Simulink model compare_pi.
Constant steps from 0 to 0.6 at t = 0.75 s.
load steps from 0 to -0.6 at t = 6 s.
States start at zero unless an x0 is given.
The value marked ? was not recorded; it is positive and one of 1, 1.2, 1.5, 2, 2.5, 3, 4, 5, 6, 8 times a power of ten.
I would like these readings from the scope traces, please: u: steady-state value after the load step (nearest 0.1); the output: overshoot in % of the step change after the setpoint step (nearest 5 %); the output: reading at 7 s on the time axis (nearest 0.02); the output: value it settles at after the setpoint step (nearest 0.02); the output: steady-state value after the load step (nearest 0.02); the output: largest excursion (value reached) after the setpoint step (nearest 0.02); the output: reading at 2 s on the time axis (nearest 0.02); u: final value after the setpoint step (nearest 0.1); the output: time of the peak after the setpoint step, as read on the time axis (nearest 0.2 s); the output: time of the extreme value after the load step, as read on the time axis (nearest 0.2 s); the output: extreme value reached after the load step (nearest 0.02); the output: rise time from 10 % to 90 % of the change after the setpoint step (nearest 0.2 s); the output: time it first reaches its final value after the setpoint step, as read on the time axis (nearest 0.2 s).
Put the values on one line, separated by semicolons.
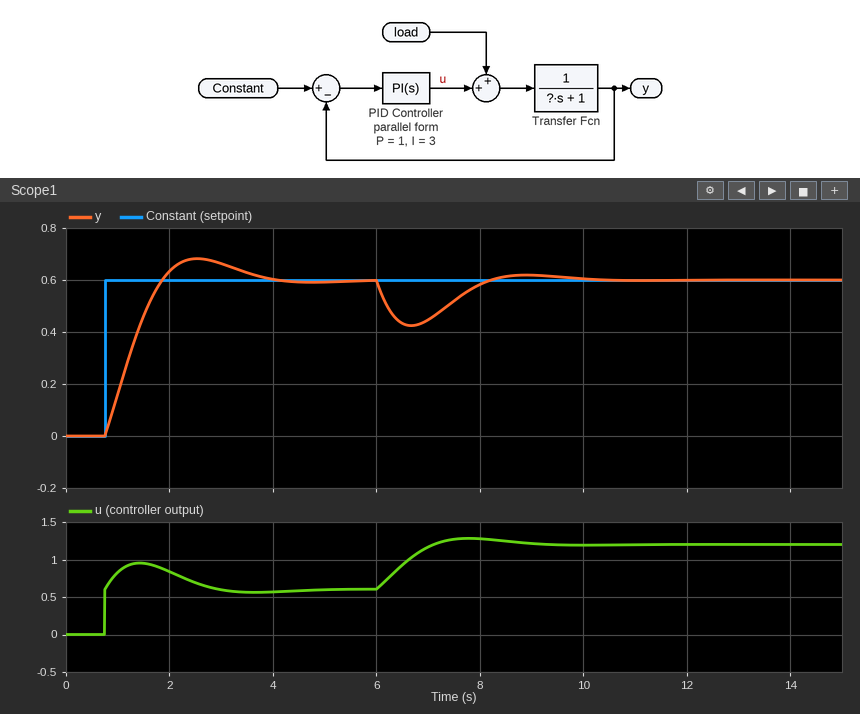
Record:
1.2; 15 %; 0.44; 0.60; 0.60; 0.68; 0.64; 0.6; 2.6 s; 6.6 s; 0.42; 0.8 s; 1.8 s
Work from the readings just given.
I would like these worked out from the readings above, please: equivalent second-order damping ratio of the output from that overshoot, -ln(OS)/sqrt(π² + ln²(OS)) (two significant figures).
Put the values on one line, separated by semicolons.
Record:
0.52
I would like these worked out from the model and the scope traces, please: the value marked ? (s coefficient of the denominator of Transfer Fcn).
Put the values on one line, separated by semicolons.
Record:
1
